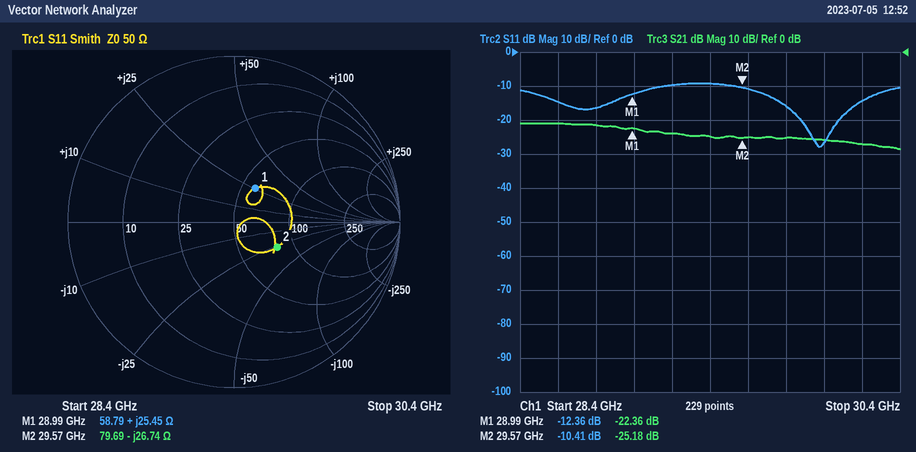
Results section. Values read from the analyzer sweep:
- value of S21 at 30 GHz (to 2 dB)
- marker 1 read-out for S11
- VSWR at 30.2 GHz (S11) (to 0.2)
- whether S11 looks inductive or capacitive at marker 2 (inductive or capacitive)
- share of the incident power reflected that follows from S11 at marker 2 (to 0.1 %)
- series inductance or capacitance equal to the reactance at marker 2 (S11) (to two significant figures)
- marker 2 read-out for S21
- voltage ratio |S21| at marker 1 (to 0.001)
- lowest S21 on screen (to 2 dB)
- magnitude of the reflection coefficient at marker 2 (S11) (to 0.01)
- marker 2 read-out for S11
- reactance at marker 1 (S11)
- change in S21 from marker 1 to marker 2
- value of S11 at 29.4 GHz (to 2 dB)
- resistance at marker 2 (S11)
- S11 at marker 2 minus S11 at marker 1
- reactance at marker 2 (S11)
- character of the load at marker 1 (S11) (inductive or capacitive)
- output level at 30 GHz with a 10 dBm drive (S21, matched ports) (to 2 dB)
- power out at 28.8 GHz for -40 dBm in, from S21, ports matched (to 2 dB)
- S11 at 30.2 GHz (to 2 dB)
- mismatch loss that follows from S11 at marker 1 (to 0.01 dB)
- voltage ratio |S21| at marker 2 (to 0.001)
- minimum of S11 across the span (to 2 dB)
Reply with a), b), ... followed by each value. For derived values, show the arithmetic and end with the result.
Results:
a) -26 dB
b) -12.36 dB
c) |Γ| = 10^(-14/20) = 0.1995; VSWR = (1 + 0.1995)/(1 − 0.1995) ≈ 1.50, so 1.4 to the nearest 0.2
d) capacitive
e) 10^(-10.41/10) ≈ 9.1 %
f) C = 1/(2π × 29.57 GHz × 26.74 Ω) ≈ 201 fF, so 200 fF to two significant figures
g) -25.18 dB
h) 10^(-22.36/20) ≈ 0.076
i) -28 dB
j) 0.30
k) -10.41 dB
l) +25.45 Ω
m) -25.18 − (-22.36) = -2.82 dB
n) -10 dB
o) 79.69 Ω
p) -10.41 − (-12.36) = 1.95 dB
q) -26.74 Ω
r) inductive
s) 10 dBm + (-26 dB) = -16 dBm
t) -40 dBm + (-22 dB) = -62 dBm
u) -14 dB
v) −10 log10(1 − 10^(-12.36/10)) ≈ 0.26 dB
w) 10^(-25.18/20) ≈ 0.055
x) -28 dB
